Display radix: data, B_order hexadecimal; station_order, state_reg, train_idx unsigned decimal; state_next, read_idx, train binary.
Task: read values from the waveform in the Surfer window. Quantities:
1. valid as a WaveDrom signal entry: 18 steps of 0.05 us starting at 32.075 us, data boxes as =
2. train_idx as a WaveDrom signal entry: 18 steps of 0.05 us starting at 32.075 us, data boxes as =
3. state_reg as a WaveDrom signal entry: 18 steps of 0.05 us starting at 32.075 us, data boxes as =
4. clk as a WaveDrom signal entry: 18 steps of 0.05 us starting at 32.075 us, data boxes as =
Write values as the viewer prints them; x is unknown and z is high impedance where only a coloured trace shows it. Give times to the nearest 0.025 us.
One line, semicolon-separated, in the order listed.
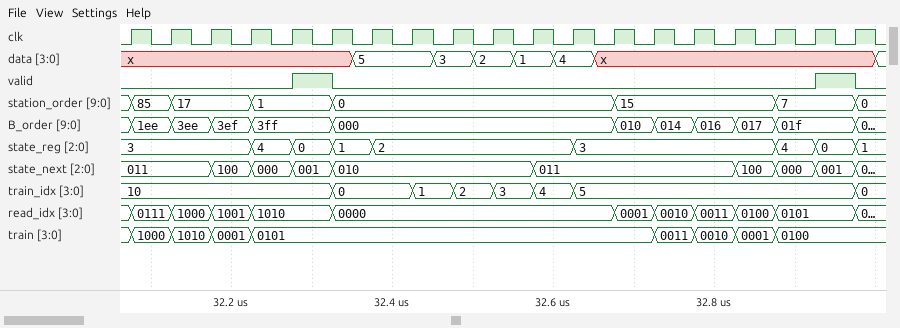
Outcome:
{name: 'valid', wave: '0...10...........1'}; {name: 'train_idx', wave: '=....=.=====......', data: '10 0 1 2 3 4 5'}; {name: 'state_reg', wave: '=..====....=....==', data: '3 4 0 1 2 3 4 0'}; {name: 'clk', wave: 'p.................'}
